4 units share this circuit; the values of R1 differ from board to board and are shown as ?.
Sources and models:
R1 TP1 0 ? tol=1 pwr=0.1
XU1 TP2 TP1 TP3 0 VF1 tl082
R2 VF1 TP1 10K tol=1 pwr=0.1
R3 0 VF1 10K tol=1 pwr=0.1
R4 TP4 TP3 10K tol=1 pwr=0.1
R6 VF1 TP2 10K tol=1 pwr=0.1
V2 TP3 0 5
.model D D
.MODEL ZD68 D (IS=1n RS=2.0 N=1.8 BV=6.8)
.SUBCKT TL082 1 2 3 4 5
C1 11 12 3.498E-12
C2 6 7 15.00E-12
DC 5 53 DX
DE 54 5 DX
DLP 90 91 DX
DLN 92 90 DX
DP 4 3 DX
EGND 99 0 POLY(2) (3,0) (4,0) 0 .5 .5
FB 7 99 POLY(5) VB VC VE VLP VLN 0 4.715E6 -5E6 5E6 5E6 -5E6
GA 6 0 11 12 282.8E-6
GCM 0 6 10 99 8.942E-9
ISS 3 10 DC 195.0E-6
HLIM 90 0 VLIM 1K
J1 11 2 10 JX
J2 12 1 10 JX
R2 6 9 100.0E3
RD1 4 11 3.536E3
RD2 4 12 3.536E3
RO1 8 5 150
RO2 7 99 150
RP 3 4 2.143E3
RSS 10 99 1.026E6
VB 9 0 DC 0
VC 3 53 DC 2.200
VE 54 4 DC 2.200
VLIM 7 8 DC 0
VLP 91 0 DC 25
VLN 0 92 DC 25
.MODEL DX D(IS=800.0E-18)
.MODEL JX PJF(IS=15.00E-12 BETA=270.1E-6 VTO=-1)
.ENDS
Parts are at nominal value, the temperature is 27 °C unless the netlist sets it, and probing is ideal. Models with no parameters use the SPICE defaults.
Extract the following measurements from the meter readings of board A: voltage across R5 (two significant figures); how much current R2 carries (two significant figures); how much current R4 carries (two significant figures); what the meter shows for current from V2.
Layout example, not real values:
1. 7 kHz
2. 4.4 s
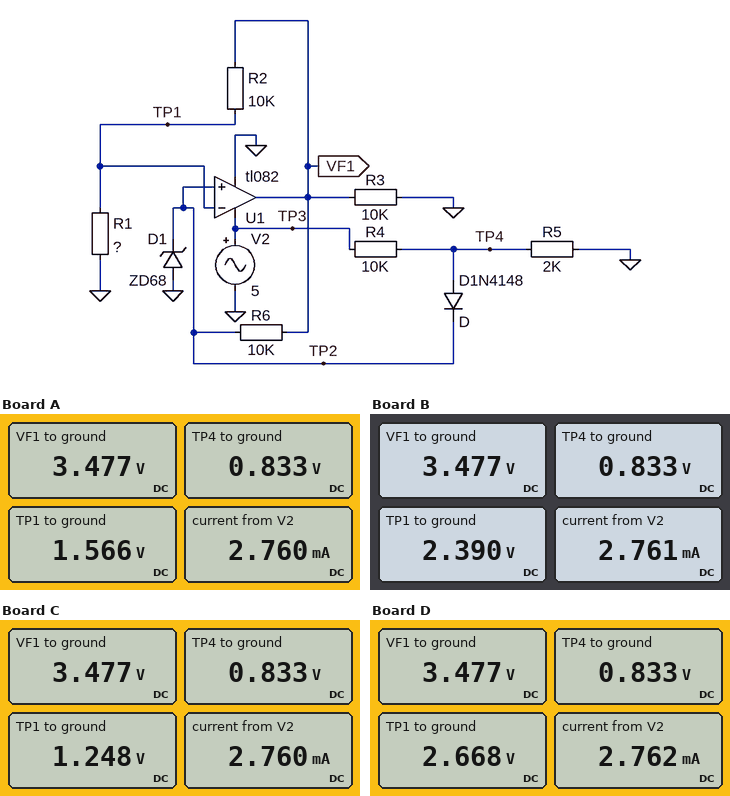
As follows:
1. 830 mV
2. 190 µA
3. 420 µA
4. 2.760 mA
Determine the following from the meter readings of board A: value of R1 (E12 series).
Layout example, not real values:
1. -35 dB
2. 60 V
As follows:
1. 8.2 kΩ
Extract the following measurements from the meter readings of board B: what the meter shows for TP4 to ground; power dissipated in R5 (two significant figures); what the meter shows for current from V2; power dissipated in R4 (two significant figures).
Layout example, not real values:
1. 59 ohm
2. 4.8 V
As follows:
1. 0.833 V
2. 350 µW
3. 2.761 mA
4. 1.7 mW
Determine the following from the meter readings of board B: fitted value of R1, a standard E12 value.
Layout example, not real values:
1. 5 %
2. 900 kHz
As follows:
1. 22 kΩ
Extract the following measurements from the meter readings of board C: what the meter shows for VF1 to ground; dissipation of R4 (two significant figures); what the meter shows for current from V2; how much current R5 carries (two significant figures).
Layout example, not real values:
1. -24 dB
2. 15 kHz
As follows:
1. 3.477 V
2. 1.7 mW
3. 2.760 mA
4. 420 µA
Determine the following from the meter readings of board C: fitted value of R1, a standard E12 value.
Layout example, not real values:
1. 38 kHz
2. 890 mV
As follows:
1. 5.6 kΩ
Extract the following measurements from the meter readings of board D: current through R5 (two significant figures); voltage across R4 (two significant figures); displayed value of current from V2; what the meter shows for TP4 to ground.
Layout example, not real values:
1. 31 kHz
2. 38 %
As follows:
1. 420 µA
2. 4.2 V
3. 2.762 mA
4. 0.833 V
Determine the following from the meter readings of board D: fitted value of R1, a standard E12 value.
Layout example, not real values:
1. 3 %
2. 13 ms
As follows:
1. 33 kΩ
